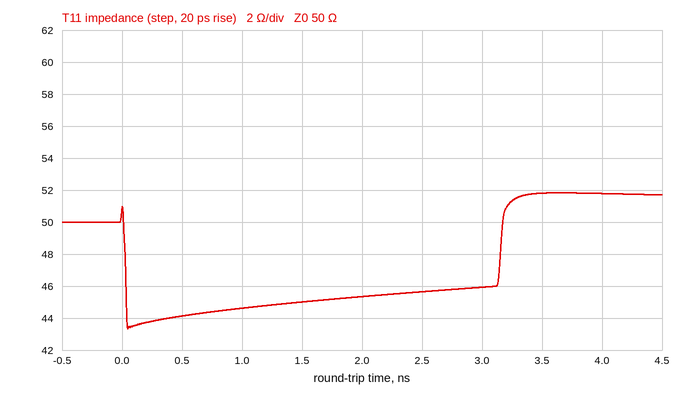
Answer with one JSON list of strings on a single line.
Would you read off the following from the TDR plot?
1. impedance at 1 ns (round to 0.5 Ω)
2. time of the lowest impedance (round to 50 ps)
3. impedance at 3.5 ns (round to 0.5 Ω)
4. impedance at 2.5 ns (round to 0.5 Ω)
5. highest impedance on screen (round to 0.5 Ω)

["44.5 Ω", "50 ps", "52.0 Ω", "45.5 Ω", "52.0 Ω"]
